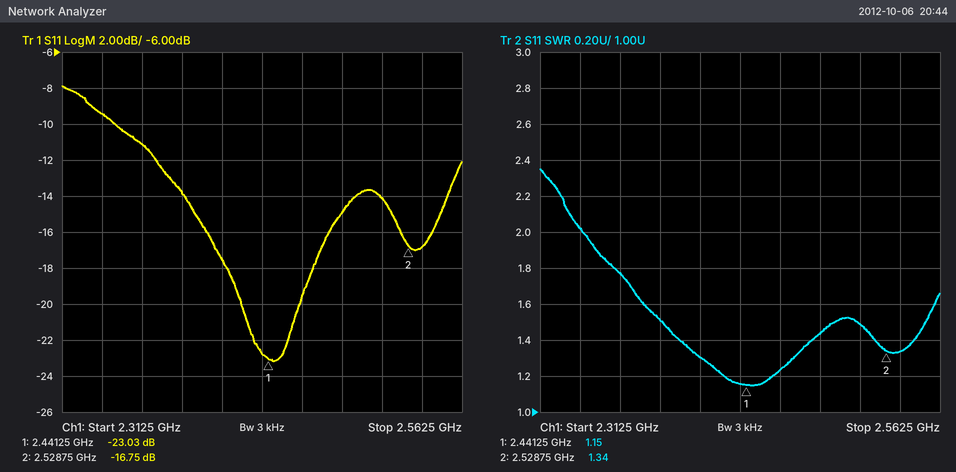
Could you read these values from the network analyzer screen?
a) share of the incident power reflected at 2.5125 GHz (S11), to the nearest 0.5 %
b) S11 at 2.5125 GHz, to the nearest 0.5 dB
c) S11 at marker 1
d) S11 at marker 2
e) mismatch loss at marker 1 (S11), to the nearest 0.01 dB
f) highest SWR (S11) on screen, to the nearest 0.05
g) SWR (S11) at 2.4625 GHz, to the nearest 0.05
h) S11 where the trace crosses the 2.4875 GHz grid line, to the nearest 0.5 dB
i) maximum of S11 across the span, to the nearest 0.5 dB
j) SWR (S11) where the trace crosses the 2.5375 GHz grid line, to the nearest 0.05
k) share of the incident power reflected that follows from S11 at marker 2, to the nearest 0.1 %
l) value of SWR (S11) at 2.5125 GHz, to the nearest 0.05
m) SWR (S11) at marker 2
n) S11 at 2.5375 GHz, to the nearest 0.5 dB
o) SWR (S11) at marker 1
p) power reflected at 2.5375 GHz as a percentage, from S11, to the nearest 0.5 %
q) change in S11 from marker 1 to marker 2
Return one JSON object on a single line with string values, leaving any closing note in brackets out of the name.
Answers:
{"share of the incident power reflected at 2.5125 GHz (S11), to the nearest 0.5 %": "4.0 %", "S11 at 2.5125 GHz, to the nearest 0.5 dB": "-14.0 dB", "S11 at marker 1": "-23.03 dB", "S11 at marker 2": "-16.75 dB", "mismatch loss at marker 1 (S11), to the nearest 0.01 dB": "0.02 dB", "highest SWR (S11) on screen, to the nearest 0.05": "2.35", "SWR (S11) at 2.4625 GHz, to the nearest 0.05": "1.25", "S11 where the trace crosses the 2.4875 GHz grid line, to the nearest 0.5 dB": "-15.0 dB", "maximum of S11 across the span, to the nearest 0.5 dB": "-8.0 dB", "SWR (S11) where the trace crosses the 2.5375 GHz grid line, to the nearest 0.05": "1.35", "share of the incident power reflected that follows from S11 at marker 2, to the nearest 0.1 %": "2.1 %", "value of SWR (S11) at 2.5125 GHz, to the nearest 0.05": "1.50", "SWR (S11) at marker 2": "1.34", "S11 at 2.5375 GHz, to the nearest 0.5 dB": "-17.0 dB", "SWR (S11) at marker 1": "1.15", "power reflected at 2.5375 GHz as a percentage, from S11, to the nearest 0.5 %": "2.0 %", "change in S11 from marker 1 to marker 2": "6.28 dB"}
